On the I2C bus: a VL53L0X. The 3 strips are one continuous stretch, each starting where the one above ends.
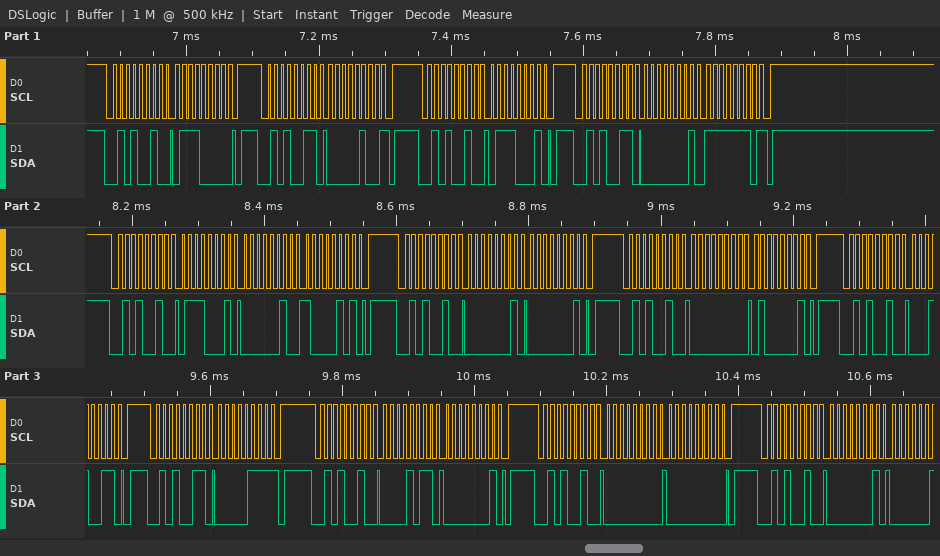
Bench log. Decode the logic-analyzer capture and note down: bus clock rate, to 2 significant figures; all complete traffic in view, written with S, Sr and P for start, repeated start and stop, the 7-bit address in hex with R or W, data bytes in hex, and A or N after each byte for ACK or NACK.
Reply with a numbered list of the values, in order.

1. 100 kHz
2. S 29W A 70 A P S 29R A 04 N P S 29W A 71 A P S 29R A 01 A FE N P S 29W A 71 A 02 A 85 A P S 29W A 01 A 01 A P S 29W A 00 A 41 A P S 29W A 13 A P S 29R A 07 N P S 29W A 0B A 01 A P S 29W A 00 A 00 A P S 29W A 01 A
